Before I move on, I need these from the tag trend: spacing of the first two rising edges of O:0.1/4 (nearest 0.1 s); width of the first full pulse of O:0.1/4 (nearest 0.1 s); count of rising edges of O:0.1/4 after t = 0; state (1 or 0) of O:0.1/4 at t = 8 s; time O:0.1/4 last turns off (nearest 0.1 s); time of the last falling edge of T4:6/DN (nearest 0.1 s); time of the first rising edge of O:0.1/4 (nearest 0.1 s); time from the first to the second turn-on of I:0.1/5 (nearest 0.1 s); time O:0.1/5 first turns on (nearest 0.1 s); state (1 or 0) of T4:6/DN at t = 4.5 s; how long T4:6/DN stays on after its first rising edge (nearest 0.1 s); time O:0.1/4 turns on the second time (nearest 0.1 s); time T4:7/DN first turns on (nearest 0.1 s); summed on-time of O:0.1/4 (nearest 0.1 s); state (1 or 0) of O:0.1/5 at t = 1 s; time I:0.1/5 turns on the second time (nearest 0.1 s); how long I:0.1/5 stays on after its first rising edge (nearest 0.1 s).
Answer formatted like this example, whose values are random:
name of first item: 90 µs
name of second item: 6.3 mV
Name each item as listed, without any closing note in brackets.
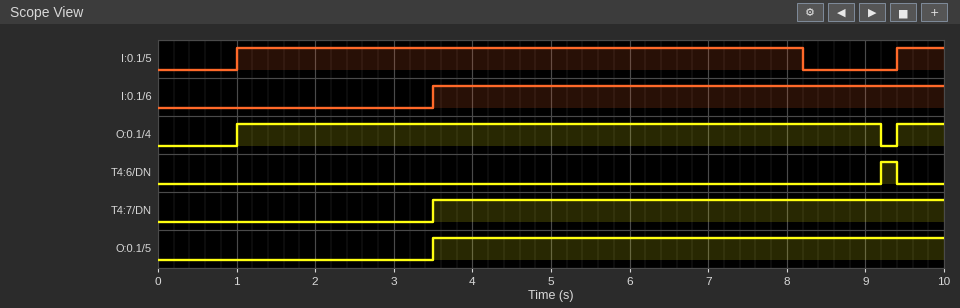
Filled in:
spacing of the first two rising edges of O:0.1/4: 8.4 s
width of the first full pulse of O:0.1/4: 8.2 s
count of rising edges of O:0.1/4 after t = 0: 2
state (1 or 0) of O:0.1/4 at t = 8 s: 1
time O:0.1/4 last turns off: 9.2 s
time of the last falling edge of T4:6/DN: 9.4 s
time of the first rising edge of O:0.1/4: 1.0 s
time from the first to the second turn-on of I:0.1/5: 8.4 s
time O:0.1/5 first turns on: 3.5 s
state (1 or 0) of T4:6/DN at t = 4.5 s: 0
how long T4:6/DN stays on after its first rising edge: 0.2 s
time O:0.1/4 turns on the second time: 9.4 s
time T4:7/DN first turns on: 3.5 s
summed on-time of O:0.1/4: 8.8 s
state (1 or 0) of O:0.1/5 at t = 1 s: 0
time I:0.1/5 turns on the second time: 9.4 s
how long I:0.1/5 stays on after its first rising edge: 7.2 s
